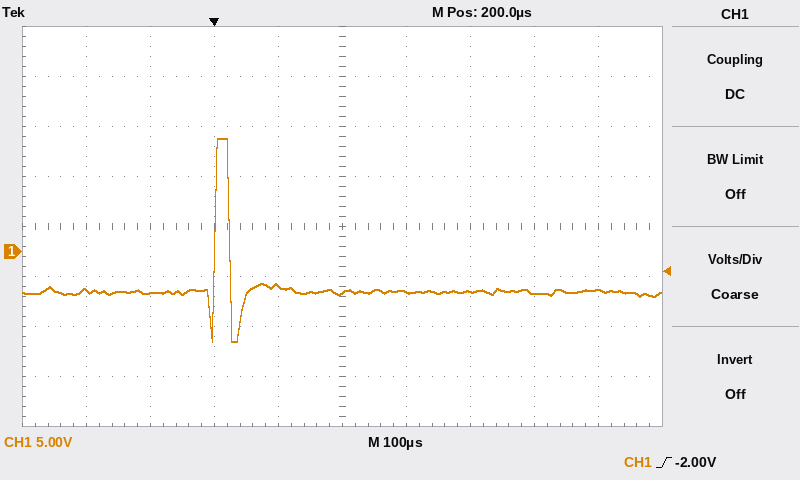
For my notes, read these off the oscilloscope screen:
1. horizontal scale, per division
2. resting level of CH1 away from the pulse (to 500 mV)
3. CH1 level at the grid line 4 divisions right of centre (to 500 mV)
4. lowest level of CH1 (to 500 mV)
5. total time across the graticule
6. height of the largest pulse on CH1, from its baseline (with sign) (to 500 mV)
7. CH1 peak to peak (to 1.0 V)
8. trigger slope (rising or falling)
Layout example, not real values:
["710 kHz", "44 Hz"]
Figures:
["100 µs", "-4.0 V", "-4.0 V", "-9.0 V", "1 ms", "+15.5 V", "20.0 V", "rising"]
